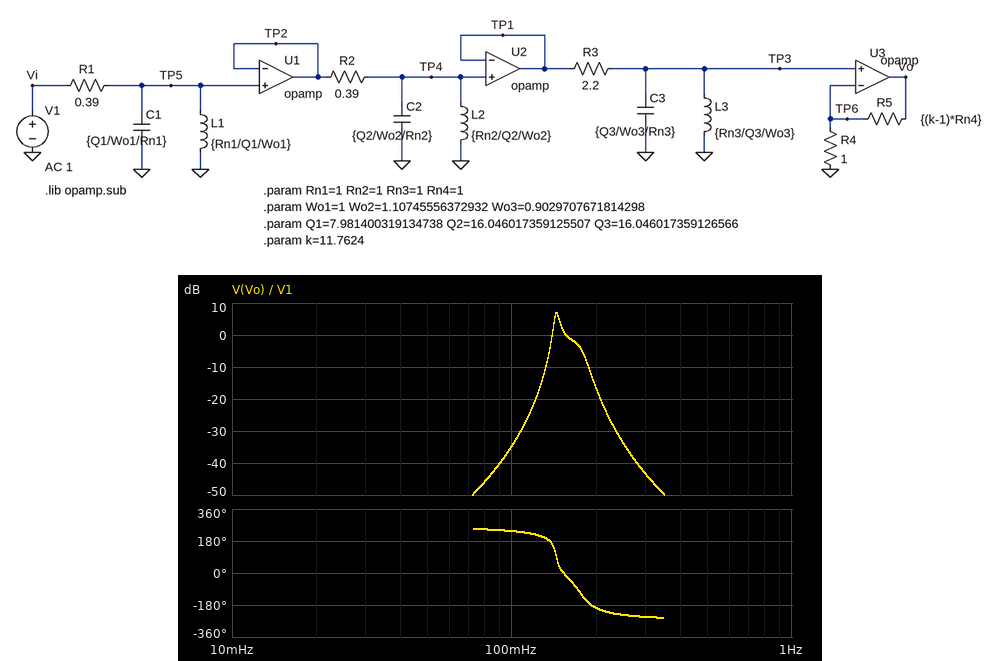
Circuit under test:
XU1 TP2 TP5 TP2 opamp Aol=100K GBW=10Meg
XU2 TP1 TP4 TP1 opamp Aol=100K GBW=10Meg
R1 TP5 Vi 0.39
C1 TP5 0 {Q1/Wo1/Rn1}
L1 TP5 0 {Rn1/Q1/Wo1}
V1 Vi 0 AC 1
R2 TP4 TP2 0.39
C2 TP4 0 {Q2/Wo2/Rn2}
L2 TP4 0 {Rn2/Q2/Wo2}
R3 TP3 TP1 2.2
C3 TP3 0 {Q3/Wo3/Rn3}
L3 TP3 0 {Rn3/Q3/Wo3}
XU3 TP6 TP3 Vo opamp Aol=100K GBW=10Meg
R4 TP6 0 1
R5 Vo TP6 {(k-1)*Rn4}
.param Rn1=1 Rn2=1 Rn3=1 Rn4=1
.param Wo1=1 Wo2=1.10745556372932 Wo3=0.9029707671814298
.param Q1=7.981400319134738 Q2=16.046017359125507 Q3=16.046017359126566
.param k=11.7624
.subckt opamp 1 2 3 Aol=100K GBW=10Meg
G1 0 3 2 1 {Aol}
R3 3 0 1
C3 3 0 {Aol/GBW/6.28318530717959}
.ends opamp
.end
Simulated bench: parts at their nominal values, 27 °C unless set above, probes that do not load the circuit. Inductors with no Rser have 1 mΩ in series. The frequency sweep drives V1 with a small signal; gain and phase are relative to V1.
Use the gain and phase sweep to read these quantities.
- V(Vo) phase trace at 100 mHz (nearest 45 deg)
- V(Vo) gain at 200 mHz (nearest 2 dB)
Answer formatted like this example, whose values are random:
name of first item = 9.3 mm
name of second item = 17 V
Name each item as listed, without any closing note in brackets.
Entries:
V(Vo) phase trace at 100 mHz = 225 deg
V(Vo) gain at 200 mHz = -16 dB
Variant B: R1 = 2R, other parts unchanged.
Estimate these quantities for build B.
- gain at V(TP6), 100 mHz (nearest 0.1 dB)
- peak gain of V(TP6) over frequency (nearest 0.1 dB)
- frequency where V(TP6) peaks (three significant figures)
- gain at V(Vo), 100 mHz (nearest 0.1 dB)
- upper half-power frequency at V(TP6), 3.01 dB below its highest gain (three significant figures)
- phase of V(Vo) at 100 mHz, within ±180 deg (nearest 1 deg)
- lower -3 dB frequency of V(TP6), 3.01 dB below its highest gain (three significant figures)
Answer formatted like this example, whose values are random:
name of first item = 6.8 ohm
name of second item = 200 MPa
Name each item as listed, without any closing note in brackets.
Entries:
gain at V(TP6), 100 mHz = -69.7 dB
peak gain of V(TP6) over frequency = -22.9 dB
frequency where V(TP6) peaks = 158 mHz
gain at V(Vo), 100 mHz = -48.3 dB
upper half-power frequency at V(TP6), 3.01 dB below its highest gain = 164 mHz
phase of V(Vo) at 100 mHz, within ±180 deg = -110 deg
lower -3 dB frequency of V(TP6), 3.01 dB below its highest gain = 142 mHz
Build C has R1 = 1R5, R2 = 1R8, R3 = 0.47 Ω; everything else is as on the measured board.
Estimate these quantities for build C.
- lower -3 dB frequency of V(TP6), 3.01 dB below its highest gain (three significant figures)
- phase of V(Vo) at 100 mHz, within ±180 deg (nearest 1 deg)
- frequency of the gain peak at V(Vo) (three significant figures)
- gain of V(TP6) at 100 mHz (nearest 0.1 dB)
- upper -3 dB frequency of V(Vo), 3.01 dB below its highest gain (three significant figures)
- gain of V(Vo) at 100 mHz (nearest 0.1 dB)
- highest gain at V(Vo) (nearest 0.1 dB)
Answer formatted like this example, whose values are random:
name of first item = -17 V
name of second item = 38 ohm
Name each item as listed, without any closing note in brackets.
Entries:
lower -3 dB frequency of V(TP6), 3.01 dB below its highest gain = 153 mHz
phase of V(Vo) at 100 mHz, within ±180 deg = -113 deg
frequency of the gain peak at V(Vo) = 175 mHz
gain of V(TP6) at 100 mHz = -67.2 dB
upper -3 dB frequency of V(Vo), 3.01 dB below its highest gain = 179 mHz
gain of V(Vo) at 100 mHz = -45.8 dB
highest gain at V(Vo) = -0.3 dB
